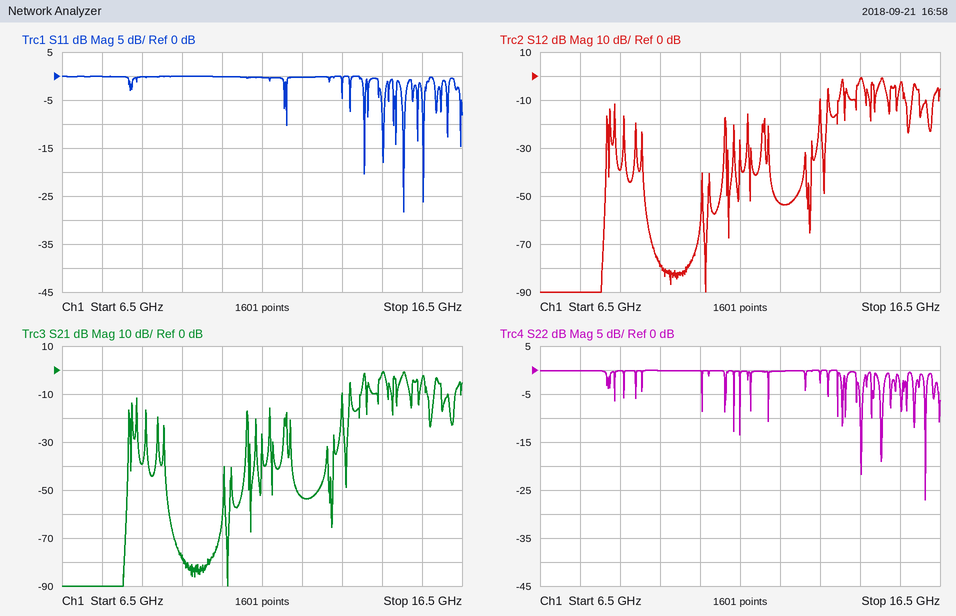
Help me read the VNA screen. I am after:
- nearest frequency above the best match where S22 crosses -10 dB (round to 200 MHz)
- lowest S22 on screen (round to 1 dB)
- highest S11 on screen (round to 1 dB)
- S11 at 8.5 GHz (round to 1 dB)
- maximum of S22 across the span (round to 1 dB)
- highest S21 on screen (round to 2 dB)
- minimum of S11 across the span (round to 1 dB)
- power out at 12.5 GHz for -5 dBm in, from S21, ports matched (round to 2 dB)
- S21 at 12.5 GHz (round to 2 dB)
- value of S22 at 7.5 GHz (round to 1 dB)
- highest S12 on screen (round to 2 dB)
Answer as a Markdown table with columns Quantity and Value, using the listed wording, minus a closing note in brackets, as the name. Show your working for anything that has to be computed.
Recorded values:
| Quantity | Value |
|---|---|
| nearest frequency above the best match where S22 crosses -10 dB | 16.2 GHz |
| lowest S22 on screen | -27 dB |
| highest S11 on screen | 0 dB |
| S11 at 8.5 GHz | 0 dB |
| maximum of S22 across the span | 0 dB |
| highest S21 on screen | 0 dB |
| minimum of S11 across the span | -28 dB |
| power out at 12.5 GHz for -5 dBm in, from S21, ports matched | -5 dBm + (-54 dB) = -58 dBm |
| S21 at 12.5 GHz | -54 dB |
| value of S22 at 7.5 GHz | 0 dB |
| highest S12 on screen | 0 dB |
